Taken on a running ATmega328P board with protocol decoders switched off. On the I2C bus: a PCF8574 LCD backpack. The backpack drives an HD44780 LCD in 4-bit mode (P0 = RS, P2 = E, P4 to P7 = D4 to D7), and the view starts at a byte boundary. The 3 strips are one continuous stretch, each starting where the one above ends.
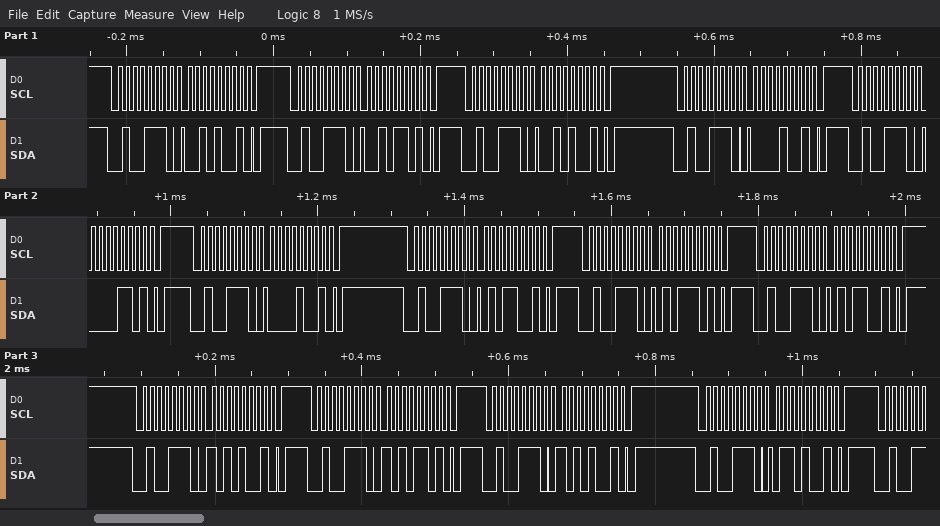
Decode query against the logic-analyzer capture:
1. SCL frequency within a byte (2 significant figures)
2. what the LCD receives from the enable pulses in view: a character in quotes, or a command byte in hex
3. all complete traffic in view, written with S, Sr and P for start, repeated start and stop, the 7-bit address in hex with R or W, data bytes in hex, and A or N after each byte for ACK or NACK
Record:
100 kHz
' ' 'Z'
S 27W A 29 A P S 27W A 2D A P S 27W A 29 A P S 27W A 09 A P S 27W A 0D A P S 27W A 09 A P S 27W A 59 A P S 27W A 5D A P S 27W A 59 A P S 27W A A9 A P S 27W A AD A P S 27W A A9 A P S 27W A 69 A P
